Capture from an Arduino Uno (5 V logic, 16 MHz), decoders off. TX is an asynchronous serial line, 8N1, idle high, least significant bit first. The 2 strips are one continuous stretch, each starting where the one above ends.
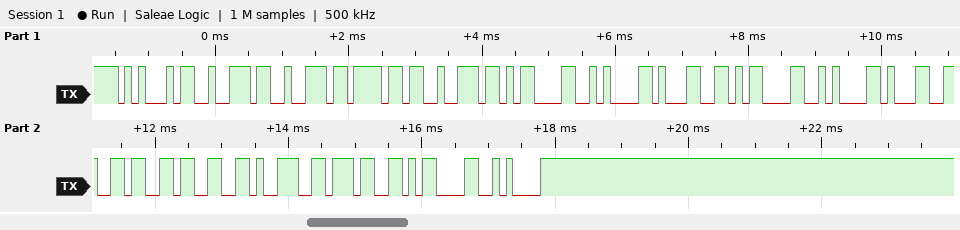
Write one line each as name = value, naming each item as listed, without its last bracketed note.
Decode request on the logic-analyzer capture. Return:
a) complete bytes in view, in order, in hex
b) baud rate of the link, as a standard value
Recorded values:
complete bytes in view, in order, in hex = 45 72 72 6F 72 0D 0A 31 0D 0A 31 36 33 39 37 0D 0A
baud rate of the link, as a standard value = 9600 baud
